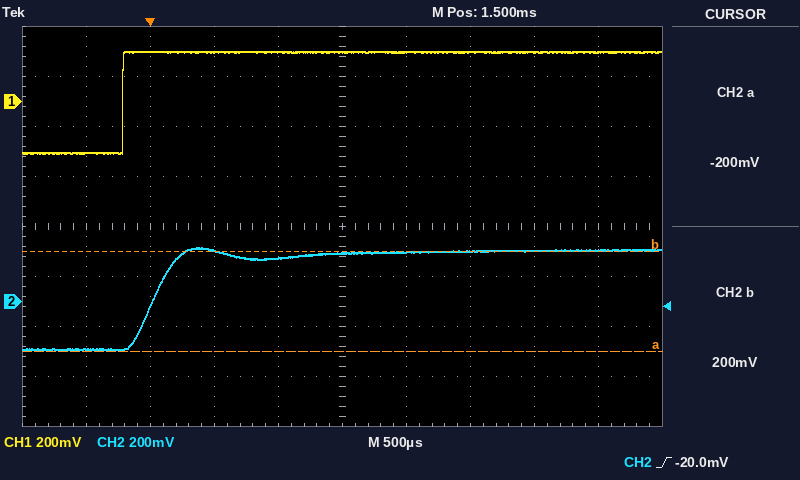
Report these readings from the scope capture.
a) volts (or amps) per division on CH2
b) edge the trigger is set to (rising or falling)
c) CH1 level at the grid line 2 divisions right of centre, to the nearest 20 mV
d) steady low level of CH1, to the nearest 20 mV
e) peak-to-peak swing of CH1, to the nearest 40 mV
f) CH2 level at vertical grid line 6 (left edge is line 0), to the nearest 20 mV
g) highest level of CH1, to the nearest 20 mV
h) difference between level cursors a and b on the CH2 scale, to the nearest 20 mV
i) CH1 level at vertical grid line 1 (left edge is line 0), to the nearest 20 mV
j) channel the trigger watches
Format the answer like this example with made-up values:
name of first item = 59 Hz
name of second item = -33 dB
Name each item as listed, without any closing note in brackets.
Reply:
volts (or amps) per division on CH2 = 200 mV
edge the trigger is set to = rising
CH1 level at the grid line 2 divisions right of centre, to the nearest 20 mV = 200 mV
steady low level of CH1, to the nearest 20 mV = -200 mV
peak-to-peak swing of CH1, to the nearest 40 mV = 400 mV
CH2 level at vertical grid line 6 (left edge is line 0), to the nearest 20 mV = 200 mV
highest level of CH1, to the nearest 20 mV = 200 mV
difference between level cursors a and b on the CH2 scale, to the nearest 20 mV = 400 mV
CH1 level at vertical grid line 1 (left edge is line 0), to the nearest 20 mV = -200 mV
channel the trigger watches = CH2
